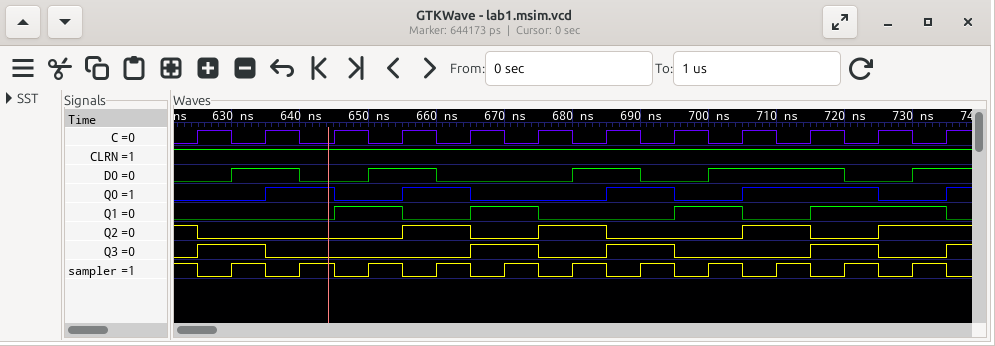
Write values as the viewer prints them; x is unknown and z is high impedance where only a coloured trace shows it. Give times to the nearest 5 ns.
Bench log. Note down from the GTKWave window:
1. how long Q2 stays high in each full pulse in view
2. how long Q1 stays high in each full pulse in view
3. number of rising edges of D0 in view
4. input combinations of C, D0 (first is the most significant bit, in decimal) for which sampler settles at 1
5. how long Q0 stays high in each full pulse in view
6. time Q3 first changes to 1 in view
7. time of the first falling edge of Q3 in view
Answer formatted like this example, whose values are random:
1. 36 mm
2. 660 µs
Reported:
1. 10 ns, 10 ns, 10 ns
2. 10 ns, 10 ns, 10 ns, 20 ns
3. 5
4. 0, 1
5. 10 ns, 10 ns, 10 ns, 20 ns
6. 625 ns
7. 635 ns
